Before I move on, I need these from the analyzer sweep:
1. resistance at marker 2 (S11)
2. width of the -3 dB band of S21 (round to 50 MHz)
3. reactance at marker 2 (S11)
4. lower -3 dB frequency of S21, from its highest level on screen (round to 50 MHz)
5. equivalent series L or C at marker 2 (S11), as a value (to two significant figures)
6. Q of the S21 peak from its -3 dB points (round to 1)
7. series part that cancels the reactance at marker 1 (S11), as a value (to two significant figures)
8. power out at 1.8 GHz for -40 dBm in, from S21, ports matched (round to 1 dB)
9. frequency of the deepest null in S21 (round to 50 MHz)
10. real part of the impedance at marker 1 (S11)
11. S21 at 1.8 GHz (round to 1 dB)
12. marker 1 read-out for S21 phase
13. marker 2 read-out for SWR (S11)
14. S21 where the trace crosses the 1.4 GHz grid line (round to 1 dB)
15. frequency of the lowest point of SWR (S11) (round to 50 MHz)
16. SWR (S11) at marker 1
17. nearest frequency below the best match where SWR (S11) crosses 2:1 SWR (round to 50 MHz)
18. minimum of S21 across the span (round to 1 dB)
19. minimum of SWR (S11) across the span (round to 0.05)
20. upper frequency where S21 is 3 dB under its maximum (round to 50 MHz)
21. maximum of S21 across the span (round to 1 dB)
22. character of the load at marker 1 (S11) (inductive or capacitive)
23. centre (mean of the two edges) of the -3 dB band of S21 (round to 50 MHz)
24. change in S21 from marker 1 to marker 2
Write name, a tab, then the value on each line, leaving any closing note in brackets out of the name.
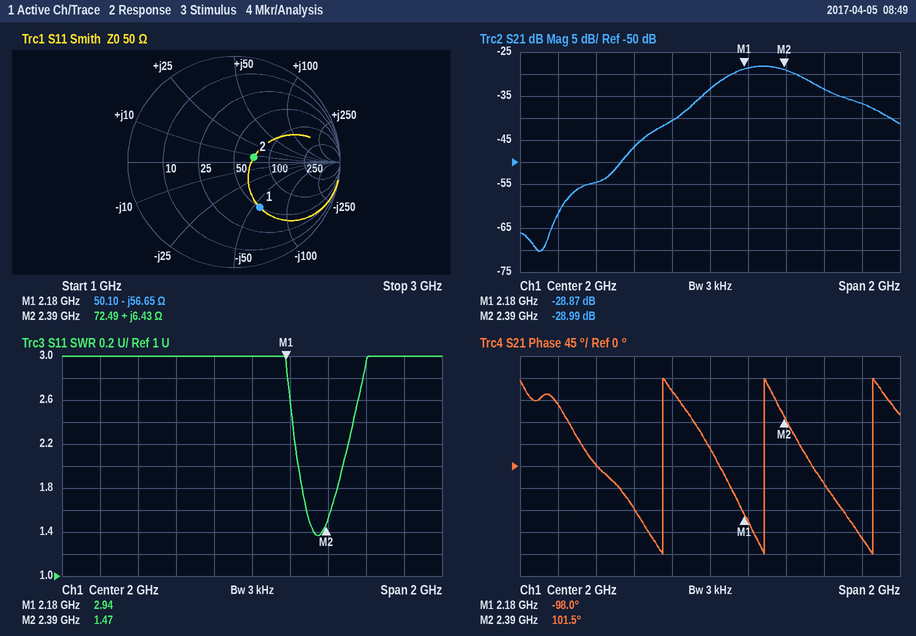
resistance at marker 2	72.49 Ω
width of the -3 dB band of S21	450 MHz
reactance at marker 2	+6.43 Ω
lower -3 dB frequency of S21, from its highest level on screen	2.05 GHz
equivalent series L or C at marker 2 (S11), as a value	430 pH
Q of the S21 peak from its -3 dB points	5
series part that cancels the reactance at marker 1 (S11), as a value	4.1 nH
power out at 1.8 GHz for -40 dBm in, from S21, ports matched	-81 dBm
frequency of the deepest null in S21	1.10 GHz
real part of the impedance at marker 1	50.10 Ω
S21 at 1.8 GHz	-41 dB
marker 1 read-out for S21 phase	-98.0°
marker 2 read-out for SWR	1.47
S21 where the trace crosses the 1.4 GHz grid line	-55 dB
frequency of the lowest point of SWR (S11)	2.35 GHz
SWR (S11) at marker 1	2.94
nearest frequency below the best match where SWR (S11) crosses 2:1 SWR	2.25 GHz
minimum of S21 across the span	-70 dB
minimum of SWR (S11) across the span	1.35
upper frequency where S21 is 3 dB under its maximum	2.50 GHz
maximum of S21 across the span	-28 dB
character of the load at marker 1 (S11)	capacitive
centre (mean of the two edges) of the -3 dB band of S21	2.30 GHz
change in S21 from marker 1 to marker 2	-0.12 dB
